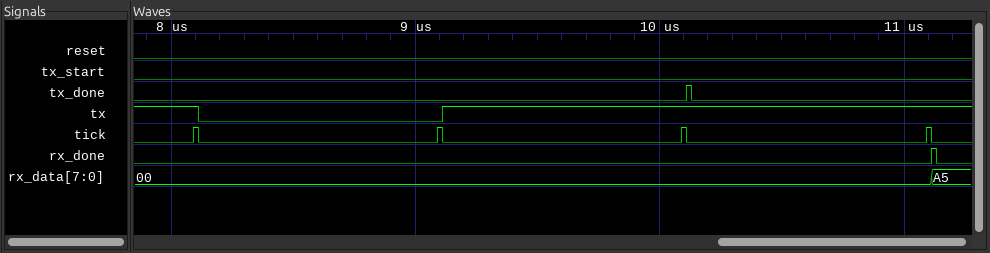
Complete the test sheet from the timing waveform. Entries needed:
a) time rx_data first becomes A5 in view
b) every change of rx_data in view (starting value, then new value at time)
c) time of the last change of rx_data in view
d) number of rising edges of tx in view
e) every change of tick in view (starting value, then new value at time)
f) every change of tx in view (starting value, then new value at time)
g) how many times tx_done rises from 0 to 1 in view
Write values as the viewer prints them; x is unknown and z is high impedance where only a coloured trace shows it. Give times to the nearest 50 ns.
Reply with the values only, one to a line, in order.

11100 ns
00, A5 at 11100 ns
11100 ns
1
0, 1 at 8100 ns, 0 at 8100 ns, 1 at 9100 ns, 0 at 9100 ns, 1 at 10100 ns, 0 at 10100 ns, 1 at 11100 ns, 0 at 11100 ns
1, 0 at 8100 ns, 1 at 9100 ns
1
